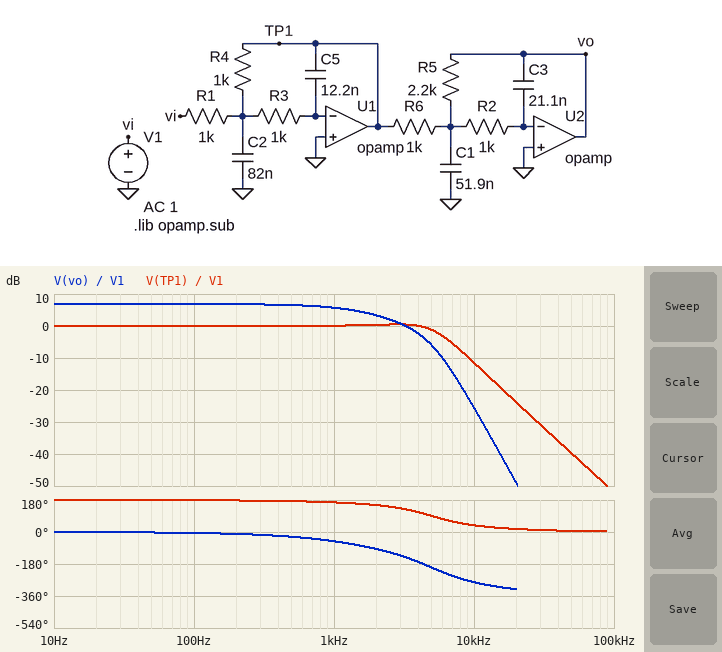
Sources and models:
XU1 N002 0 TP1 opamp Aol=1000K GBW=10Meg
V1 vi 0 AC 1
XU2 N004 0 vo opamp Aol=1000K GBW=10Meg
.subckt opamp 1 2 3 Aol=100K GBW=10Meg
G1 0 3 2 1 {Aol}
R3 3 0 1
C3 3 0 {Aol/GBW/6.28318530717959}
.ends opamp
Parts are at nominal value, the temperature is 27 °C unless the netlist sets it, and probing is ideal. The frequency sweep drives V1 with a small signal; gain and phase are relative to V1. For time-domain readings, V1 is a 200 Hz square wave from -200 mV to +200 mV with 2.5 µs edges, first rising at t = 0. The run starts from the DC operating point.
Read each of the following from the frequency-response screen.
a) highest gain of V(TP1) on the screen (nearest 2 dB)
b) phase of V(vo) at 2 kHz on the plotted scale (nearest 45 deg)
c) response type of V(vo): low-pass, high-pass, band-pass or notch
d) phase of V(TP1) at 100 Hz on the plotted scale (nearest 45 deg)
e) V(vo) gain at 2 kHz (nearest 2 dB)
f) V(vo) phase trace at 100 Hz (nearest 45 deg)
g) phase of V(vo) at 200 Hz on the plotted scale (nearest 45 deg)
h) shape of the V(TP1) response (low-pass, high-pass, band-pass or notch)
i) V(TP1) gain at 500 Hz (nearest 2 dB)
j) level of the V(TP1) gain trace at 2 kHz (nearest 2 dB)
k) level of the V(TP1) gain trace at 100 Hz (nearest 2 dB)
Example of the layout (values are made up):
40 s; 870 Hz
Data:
0 dB; -90 deg; low-pass; 180 deg; 4 dB; 0 deg; 0 deg; low-pass; 0 dB; 0 dB; 0 dB
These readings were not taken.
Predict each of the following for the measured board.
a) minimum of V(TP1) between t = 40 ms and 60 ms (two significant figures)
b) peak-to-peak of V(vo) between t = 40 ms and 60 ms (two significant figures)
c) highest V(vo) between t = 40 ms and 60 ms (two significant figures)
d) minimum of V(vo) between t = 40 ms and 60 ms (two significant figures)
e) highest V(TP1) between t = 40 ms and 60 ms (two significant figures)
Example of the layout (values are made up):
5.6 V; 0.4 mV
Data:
-250 mV; 880 mV; 440 mV; -440 mV; 250 mV
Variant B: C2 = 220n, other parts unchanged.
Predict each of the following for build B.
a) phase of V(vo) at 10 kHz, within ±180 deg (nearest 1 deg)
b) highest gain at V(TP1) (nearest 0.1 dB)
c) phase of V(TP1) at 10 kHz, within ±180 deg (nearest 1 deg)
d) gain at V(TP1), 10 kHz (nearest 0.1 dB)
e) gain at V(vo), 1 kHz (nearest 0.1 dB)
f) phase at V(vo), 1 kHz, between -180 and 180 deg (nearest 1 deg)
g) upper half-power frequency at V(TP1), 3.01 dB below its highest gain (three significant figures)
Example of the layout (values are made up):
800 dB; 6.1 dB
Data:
53 deg; 3.6 dB; 13 deg; -19.9 dB; 6.3 dB; -53 deg; 3.65 kHz
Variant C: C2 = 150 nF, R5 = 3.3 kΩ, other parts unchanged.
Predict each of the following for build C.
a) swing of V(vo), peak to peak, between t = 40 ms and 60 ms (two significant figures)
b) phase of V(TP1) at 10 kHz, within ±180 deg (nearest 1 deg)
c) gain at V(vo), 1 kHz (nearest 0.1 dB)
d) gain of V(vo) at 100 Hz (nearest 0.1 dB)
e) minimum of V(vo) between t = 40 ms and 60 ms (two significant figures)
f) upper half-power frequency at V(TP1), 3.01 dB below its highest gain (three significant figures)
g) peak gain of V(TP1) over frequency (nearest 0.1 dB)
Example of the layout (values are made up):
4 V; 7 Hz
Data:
1.3 V; 20 deg; 8.3 dB; 10.3 dB; -660 mV; 4.41 kHz; 2.2 dB
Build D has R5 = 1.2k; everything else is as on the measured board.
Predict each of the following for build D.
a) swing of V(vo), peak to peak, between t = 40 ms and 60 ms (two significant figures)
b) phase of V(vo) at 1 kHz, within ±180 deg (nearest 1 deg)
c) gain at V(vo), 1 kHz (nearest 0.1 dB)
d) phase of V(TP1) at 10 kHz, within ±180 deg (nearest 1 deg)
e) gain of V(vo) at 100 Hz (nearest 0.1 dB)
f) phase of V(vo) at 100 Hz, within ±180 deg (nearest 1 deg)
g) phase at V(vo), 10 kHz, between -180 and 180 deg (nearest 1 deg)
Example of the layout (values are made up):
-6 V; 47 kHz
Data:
490 mV; -39 deg; 1.3 dB; 38 deg; 1.6 dB; -4 deg; 85 deg
